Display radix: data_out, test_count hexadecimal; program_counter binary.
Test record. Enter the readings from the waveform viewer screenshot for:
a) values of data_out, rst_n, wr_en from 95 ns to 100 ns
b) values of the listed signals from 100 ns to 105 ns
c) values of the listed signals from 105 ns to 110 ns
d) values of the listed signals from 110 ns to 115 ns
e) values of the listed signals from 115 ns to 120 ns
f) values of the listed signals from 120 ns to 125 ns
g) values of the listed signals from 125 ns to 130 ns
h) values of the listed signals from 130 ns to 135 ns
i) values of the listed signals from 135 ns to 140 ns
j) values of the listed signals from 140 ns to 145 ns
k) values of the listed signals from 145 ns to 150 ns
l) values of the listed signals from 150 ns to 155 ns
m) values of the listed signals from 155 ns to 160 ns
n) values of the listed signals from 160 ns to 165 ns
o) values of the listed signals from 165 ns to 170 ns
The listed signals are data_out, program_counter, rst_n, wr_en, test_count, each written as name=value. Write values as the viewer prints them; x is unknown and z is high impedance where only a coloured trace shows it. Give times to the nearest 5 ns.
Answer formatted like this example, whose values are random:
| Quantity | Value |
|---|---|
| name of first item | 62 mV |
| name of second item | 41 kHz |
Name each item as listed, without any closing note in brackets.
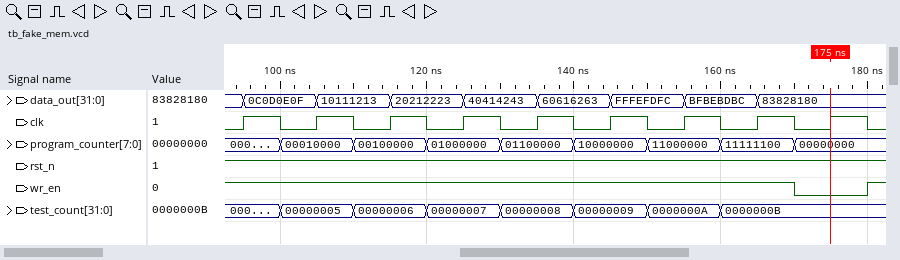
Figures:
| Quantity | Value |
|---|---|
| values of data_out, rst_n, wr_en from 95 ns to 100 ns | data_out=0C0D0E0F, rst_n=1, wr_en=1 |
| values of the listed signals from 100 ns to 105 ns | data_out=0C0D0E0F, program_counter=00010000, rst_n=1, wr_en=1, test_count=00000005 |
| values of the listed signals from 105 ns to 110 ns | data_out=10111213, program_counter=00010000, rst_n=1, wr_en=1, test_count=00000005 |
| values of the listed signals from 110 ns to 115 ns | data_out=10111213, program_counter=00100000, rst_n=1, wr_en=1, test_count=00000006 |
| values of the listed signals from 115 ns to 120 ns | data_out=20212223, program_counter=00100000, rst_n=1, wr_en=1, test_count=00000006 |
| values of the listed signals from 120 ns to 125 ns | data_out=20212223, program_counter=01000000, rst_n=1, wr_en=1, test_count=00000007 |
| values of the listed signals from 125 ns to 130 ns | data_out=40414243, program_counter=01000000, rst_n=1, wr_en=1, test_count=00000007 |
| values of the listed signals from 130 ns to 135 ns | data_out=40414243, program_counter=01100000, rst_n=1, wr_en=1, test_count=00000008 |
| values of the listed signals from 135 ns to 140 ns | data_out=60616263, program_counter=01100000, rst_n=1, wr_en=1, test_count=00000008 |
| values of the listed signals from 140 ns to 145 ns | data_out=60616263, program_counter=10000000, rst_n=1, wr_en=1, test_count=00000009 |
| values of the listed signals from 145 ns to 150 ns | data_out=FFFEFDFC, program_counter=10000000, rst_n=1, wr_en=1, test_count=00000009 |
| values of the listed signals from 150 ns to 155 ns | data_out=FFFEFDFC, program_counter=11000000, rst_n=1, wr_en=1, test_count=0000000A |
| values of the listed signals from 155 ns to 160 ns | data_out=BFBEBDBC, program_counter=11000000, rst_n=1, wr_en=1, test_count=0000000A |
| values of the listed signals from 160 ns to 165 ns | data_out=BFBEBDBC, program_counter=11111100, rst_n=1, wr_en=1, test_count=0000000B |
| values of the listed signals from 165 ns to 170 ns | data_out=83828180, program_counter=11111100, rst_n=1, wr_en=1, test_count=0000000B |
